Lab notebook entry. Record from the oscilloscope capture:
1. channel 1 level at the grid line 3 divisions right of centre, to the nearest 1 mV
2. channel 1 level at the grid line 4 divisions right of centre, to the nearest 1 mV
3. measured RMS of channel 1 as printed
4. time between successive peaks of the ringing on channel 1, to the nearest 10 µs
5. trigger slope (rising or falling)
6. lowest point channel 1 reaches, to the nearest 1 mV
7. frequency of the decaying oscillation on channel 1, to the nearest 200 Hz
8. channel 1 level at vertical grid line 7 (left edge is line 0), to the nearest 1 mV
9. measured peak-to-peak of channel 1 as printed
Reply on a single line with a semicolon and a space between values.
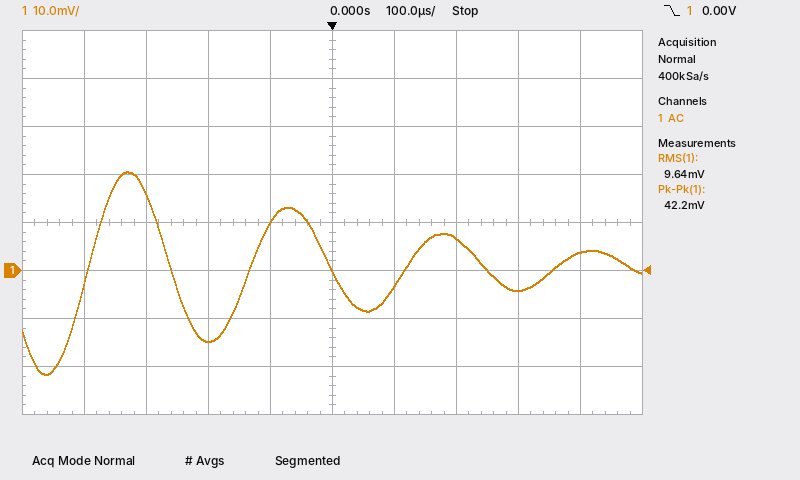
-4 mV; 4 mV; 9.64 mV; 250 µs; falling; -22 mV; 4.0 kHz; 7 mV; 42.2 mV
